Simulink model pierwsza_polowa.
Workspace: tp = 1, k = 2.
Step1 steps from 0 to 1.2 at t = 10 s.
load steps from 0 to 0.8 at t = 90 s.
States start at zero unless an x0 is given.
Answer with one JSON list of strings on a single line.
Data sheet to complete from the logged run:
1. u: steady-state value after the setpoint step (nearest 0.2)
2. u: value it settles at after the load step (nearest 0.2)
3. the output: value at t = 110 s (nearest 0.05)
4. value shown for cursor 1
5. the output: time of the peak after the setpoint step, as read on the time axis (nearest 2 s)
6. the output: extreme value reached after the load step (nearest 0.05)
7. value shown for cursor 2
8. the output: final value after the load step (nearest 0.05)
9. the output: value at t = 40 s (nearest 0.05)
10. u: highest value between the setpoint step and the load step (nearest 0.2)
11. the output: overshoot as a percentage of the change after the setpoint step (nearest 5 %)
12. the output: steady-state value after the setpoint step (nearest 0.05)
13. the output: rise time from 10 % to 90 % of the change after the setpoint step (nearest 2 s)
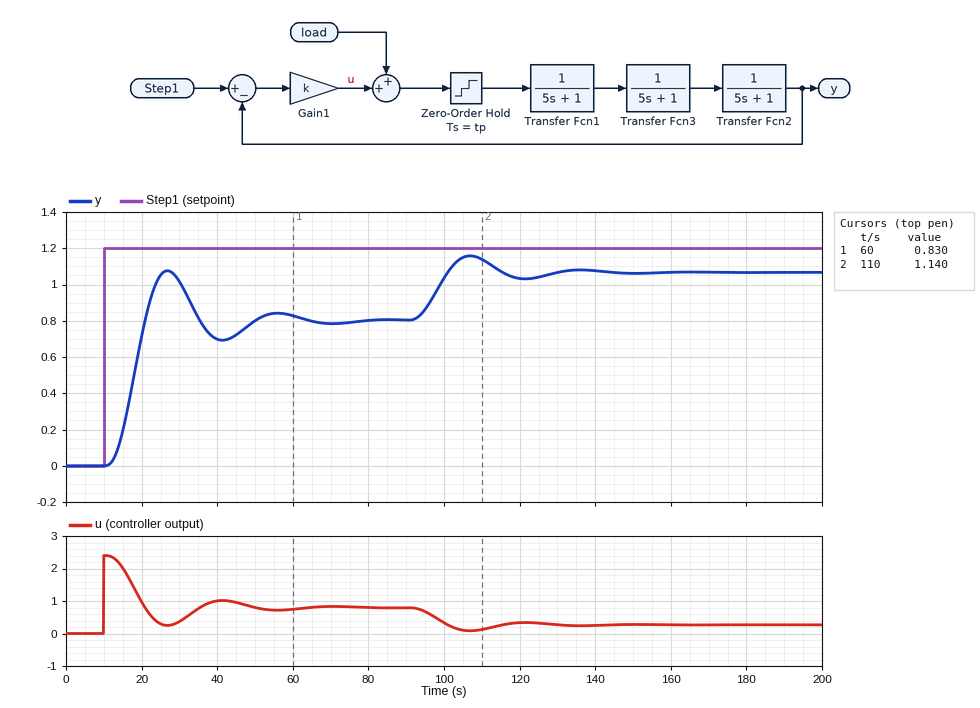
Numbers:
["0.8", "0.2", "1.15", "0.830", "26 s", "1.15", "1.140", "1.05", "0.70", "2.4", "35 %", "0.80", "6 s"]
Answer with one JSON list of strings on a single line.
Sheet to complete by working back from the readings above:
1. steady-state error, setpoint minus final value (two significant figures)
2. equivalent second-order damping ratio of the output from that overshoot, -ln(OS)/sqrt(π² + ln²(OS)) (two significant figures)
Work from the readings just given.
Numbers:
["0.40", "0.32"]
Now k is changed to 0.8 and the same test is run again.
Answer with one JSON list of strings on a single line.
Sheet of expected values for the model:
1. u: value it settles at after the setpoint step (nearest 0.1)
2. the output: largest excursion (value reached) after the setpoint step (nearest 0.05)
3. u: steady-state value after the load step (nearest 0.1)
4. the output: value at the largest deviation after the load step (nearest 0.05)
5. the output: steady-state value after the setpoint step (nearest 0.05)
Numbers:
["0.5", "0.60", "0.2", "1.05", "0.55"]
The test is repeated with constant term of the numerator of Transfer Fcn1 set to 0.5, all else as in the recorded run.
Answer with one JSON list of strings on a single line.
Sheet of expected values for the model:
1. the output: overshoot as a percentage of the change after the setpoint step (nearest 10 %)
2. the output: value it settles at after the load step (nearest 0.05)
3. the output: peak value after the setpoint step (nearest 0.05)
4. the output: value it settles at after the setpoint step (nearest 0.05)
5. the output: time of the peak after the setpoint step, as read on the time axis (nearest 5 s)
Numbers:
["20 %", "0.80", "0.70", "0.60", "30 s"]
